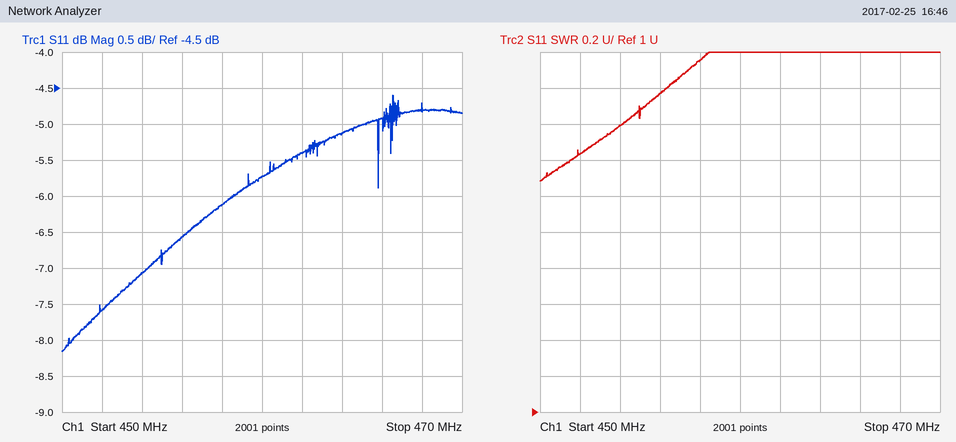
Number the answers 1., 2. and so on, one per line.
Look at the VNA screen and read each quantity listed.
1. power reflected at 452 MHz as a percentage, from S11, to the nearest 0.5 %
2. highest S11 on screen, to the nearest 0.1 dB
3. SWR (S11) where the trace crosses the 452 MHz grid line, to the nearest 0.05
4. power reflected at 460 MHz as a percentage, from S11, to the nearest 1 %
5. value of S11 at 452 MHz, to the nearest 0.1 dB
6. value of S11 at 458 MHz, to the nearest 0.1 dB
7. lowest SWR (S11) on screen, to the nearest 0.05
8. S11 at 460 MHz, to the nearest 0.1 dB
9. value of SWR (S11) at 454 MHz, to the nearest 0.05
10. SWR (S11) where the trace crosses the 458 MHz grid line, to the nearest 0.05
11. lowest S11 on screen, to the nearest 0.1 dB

1. 17.5 %
2. -4.6 dB
3. 2.45
4. 27 %
5. -7.6 dB
6. -6.1 dB
7. 2.30
8. -5.7 dB
9. 2.60
10. 2.95
11. -8.2 dB
